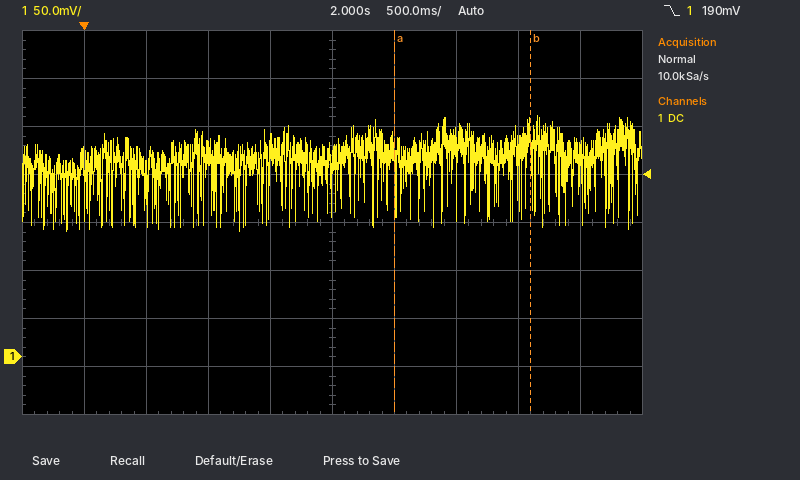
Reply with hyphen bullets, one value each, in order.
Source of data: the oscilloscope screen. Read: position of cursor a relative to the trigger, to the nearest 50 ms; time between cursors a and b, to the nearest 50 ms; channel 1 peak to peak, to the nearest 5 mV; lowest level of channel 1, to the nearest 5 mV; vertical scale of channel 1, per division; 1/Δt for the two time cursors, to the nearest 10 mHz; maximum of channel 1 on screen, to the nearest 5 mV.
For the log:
- +2.50 s
- 1.10 s
- 120 mV
- 130 mV
- 50 mV
- 910 mHz
- 250 mV
